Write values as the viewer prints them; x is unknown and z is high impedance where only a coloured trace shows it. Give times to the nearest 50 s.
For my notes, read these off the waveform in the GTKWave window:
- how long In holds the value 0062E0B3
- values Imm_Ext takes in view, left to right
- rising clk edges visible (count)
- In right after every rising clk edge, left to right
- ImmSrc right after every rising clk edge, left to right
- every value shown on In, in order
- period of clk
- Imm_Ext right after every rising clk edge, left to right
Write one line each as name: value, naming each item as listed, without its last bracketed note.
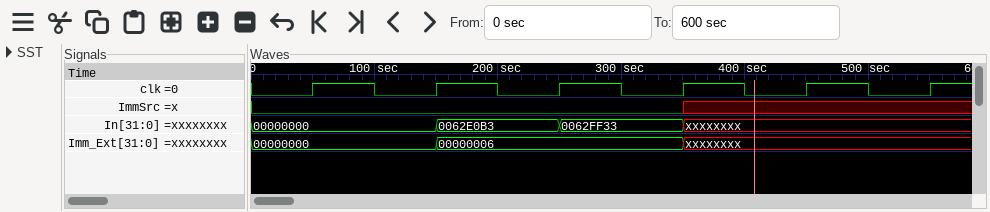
how long In holds the value 0062E0B3: 100 s
values Imm_Ext takes in view, left to right: 00000000, 00000006, xxxxxxxx
rising clk edges visible: 6
In right after every rising clk edge, left to right: 00000000, 0062E0B3, 0062FF33, xxxxxxxx, xxxxxxxx, xxxxxxxx
ImmSrc right after every rising clk edge, left to right: 0 0 0 x x x
every value shown on In, in order: 00000000, 0062E0B3, 0062FF33, xxxxxxxx
period of clk: 100 s
Imm_Ext right after every rising clk edge, left to right: 00000000, 00000006, 00000006, xxxxxxxx, xxxxxxxx, xxxxxxxx
